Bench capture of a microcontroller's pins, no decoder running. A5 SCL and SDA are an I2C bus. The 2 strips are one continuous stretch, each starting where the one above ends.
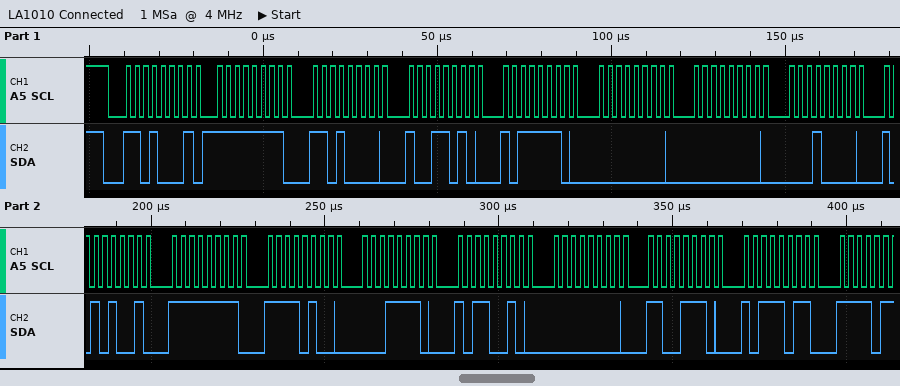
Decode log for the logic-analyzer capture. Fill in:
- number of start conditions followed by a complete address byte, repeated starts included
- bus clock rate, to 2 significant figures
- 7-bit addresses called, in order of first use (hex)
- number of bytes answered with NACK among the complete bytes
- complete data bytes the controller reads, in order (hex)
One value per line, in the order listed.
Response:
1
400 kHz
0x68
0
FF D0 9A BE 00 00 10 A9 FF F4 1E B2 00 CE BB
